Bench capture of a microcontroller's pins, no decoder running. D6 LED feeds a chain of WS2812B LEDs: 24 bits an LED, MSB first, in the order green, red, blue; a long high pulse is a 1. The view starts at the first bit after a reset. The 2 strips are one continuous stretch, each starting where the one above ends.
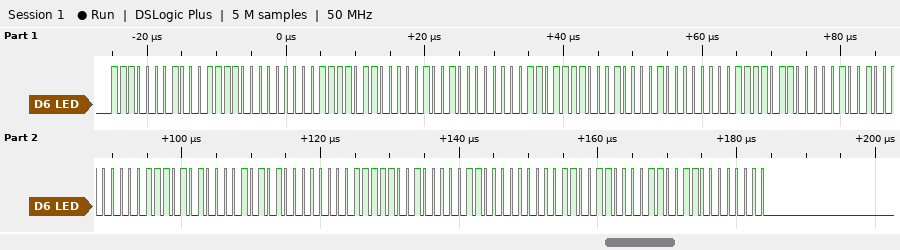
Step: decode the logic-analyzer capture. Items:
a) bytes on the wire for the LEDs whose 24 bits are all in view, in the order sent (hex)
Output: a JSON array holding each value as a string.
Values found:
["E1 1E 00 F6 09 00 DE 21 00 F6 09 00 EA 15 00 F9 06 00 CC 33 00"]
